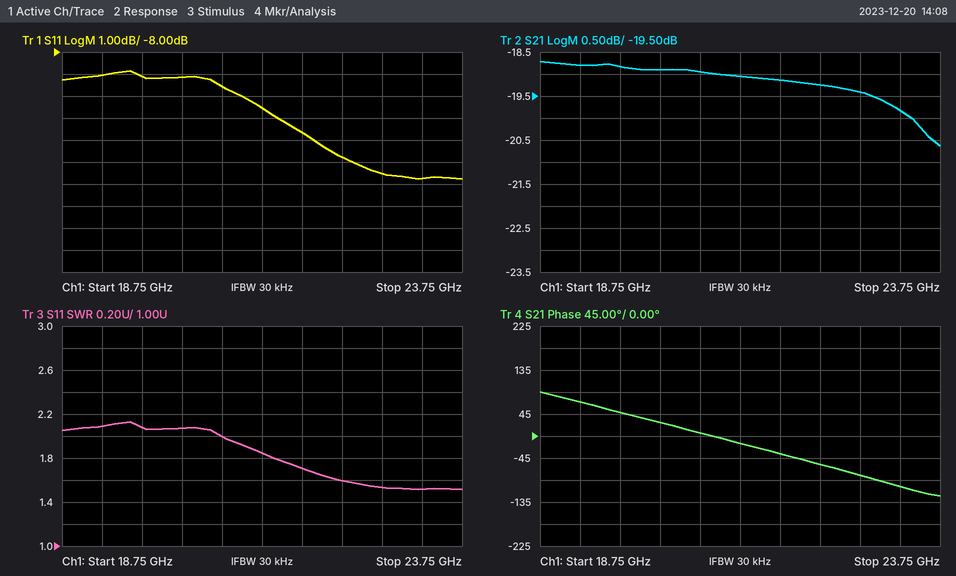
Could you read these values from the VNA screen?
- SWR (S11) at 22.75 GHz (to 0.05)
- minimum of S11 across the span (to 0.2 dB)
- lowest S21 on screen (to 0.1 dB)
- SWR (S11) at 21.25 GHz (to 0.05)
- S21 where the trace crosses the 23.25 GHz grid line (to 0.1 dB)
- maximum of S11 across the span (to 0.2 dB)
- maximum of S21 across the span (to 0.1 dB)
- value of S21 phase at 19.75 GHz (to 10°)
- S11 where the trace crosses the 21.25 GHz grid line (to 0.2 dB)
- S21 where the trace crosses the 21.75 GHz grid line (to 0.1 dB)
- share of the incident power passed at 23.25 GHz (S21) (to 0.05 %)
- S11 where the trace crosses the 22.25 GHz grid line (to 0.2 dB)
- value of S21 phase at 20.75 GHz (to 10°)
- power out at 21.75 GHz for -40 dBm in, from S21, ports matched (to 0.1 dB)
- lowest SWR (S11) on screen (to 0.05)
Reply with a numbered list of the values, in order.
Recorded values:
1. 1.55
2. -13.8 dB
3. -20.6 dB
4. 1.85
5. -19.8 dB
6. -8.8 dB
7. -18.7 dB
8. 50°
9. -10.6 dB
10. -19.1 dB
11. 1.05 %
12. -12.8 dB
13. 10°
14. -59.1 dBm
15. 1.50
